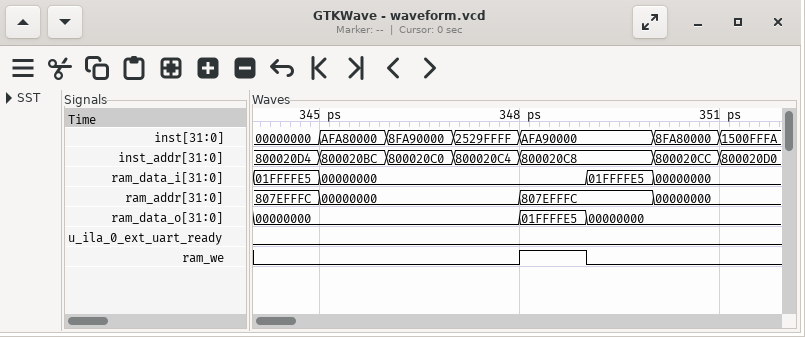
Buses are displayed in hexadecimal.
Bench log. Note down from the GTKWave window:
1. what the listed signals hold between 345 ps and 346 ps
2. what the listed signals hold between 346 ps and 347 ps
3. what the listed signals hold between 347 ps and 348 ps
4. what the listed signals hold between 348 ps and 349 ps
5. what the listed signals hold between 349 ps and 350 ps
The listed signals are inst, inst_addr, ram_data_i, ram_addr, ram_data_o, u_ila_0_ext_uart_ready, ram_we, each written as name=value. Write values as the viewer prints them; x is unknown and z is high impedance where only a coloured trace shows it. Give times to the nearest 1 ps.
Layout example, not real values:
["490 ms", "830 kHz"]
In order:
["inst=AFA80000, inst_addr=800020BC, ram_data_i=00000000, ram_addr=00000000, ram_data_o=00000000, u_ila_0_ext_uart_ready=0, ram_we=0", "inst=8FA90000, inst_addr=800020C0, ram_data_i=00000000, ram_addr=00000000, ram_data_o=00000000, u_ila_0_ext_uart_ready=0, ram_we=0", "inst=2529FFFF, inst_addr=800020C4, ram_data_i=00000000, ram_addr=00000000, ram_data_o=00000000, u_ila_0_ext_uart_ready=0, ram_we=0", "inst=AFA90000, inst_addr=800020C8, ram_data_i=00000000, ram_addr=807EFFFC, ram_data_o=01FFFFE5, u_ila_0_ext_uart_ready=0, ram_we=1", "inst=AFA90000, inst_addr=800020C8, ram_data_i=01FFFFE5, ram_addr=807EFFFC, ram_data_o=00000000, u_ila_0_ext_uart_ready=0, ram_we=0"]
